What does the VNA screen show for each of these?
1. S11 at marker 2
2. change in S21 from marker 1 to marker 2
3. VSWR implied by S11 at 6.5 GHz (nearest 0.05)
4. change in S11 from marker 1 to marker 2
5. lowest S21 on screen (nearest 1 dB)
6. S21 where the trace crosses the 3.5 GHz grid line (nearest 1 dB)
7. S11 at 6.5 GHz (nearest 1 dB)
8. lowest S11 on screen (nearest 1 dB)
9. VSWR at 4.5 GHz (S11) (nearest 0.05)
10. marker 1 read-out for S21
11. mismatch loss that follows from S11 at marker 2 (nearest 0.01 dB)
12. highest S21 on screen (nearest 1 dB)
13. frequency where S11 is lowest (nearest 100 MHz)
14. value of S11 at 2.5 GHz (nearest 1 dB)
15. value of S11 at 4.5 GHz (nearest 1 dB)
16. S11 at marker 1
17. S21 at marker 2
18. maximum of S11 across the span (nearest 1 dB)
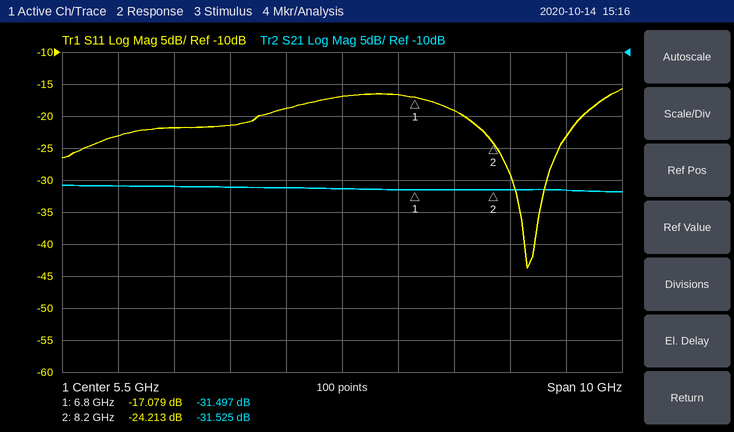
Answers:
-24.213 dB
-0.028 dB
1.35
-7.134 dB
-32 dB
-31 dB
-17 dB
-44 dB
1.25
-31.497 dB
0.02 dB
-31 dB
8.8 GHz
-22 dB
-19 dB
-17.079 dB
-31.525 dB
-16 dB
